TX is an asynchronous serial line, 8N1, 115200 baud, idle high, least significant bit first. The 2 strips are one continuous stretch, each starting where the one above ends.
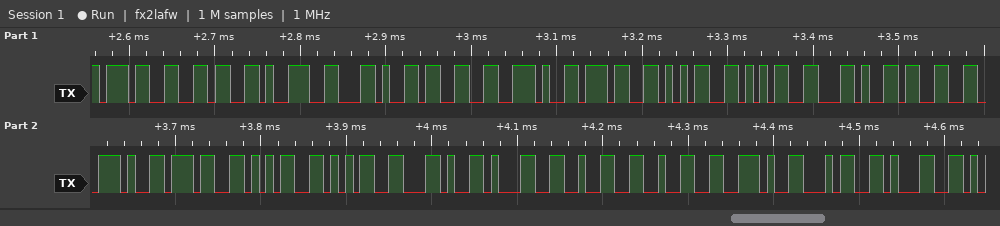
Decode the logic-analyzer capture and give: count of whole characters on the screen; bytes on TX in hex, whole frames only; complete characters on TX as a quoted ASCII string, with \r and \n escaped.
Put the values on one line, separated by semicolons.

22; 37 36 39 2C 33 2E 37 35 35 2C 33 2E 37 35 35 2C 31 32 32 2E 34 31; "769,3.755,3.755,122.41"
